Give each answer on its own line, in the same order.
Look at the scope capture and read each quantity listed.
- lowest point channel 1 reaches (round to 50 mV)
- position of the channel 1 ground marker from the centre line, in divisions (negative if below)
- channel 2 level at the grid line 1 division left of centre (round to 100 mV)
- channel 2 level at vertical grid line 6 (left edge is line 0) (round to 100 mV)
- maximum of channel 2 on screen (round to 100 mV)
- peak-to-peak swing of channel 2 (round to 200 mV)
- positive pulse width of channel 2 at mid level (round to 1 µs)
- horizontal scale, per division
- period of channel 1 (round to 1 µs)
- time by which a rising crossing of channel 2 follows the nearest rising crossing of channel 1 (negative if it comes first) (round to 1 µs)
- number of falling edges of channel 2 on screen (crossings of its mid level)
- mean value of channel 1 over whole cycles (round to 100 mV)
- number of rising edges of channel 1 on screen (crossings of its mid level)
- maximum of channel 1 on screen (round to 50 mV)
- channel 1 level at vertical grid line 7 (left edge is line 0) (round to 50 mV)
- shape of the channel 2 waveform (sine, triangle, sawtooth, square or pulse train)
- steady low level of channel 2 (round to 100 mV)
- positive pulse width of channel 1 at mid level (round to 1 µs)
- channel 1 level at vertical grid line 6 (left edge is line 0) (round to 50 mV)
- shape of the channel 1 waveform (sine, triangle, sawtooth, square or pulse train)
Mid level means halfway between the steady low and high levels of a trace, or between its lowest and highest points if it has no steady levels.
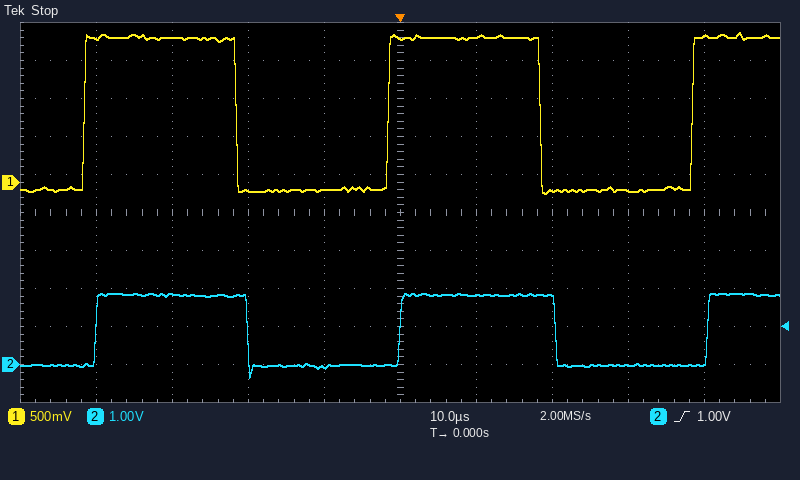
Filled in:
-150 mV
+0.8 div
-100 mV
1.8 V
1.9 V
2.2 V
20 µs
10 µs
40 µs
+2 µs
2
900 mV
3
1.95 V
-100 mV
square
0.0 V
20 µs
1.90 V
square
